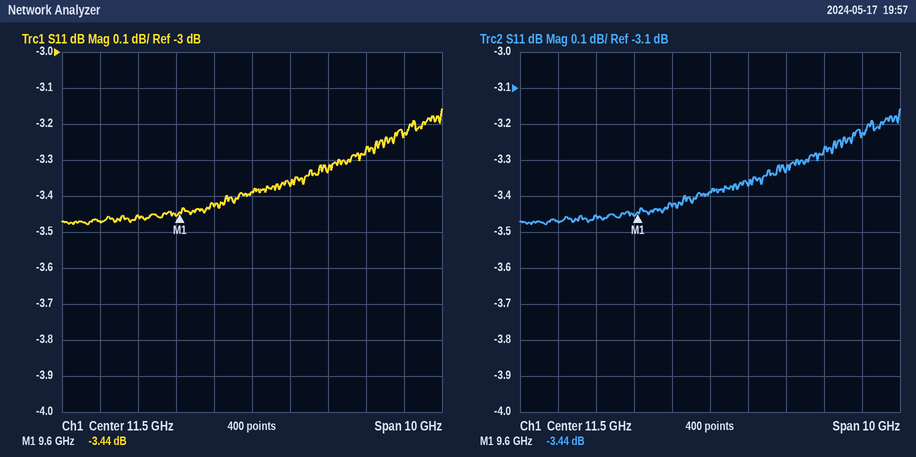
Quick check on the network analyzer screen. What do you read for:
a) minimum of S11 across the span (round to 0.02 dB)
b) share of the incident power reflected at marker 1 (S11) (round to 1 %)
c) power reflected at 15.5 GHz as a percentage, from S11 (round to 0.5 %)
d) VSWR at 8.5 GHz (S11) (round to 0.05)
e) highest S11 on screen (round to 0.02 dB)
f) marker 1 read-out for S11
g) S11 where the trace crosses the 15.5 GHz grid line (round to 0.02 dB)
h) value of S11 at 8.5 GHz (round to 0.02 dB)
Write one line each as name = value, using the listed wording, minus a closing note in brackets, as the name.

minimum of S11 across the span = -3.48 dB
share of the incident power reflected at marker 1 (S11) = 45 %
power reflected at 15.5 GHz as a percentage, from S11 = 47.5 %
VSWR at 8.5 GHz (S11) = 5.10
highest S11 on screen = -3.16 dB
marker 1 read-out for S11 = -3.44 dB
S11 where the trace crosses the 15.5 GHz grid line = -3.22 dB
value of S11 at 8.5 GHz = -3.46 dB
